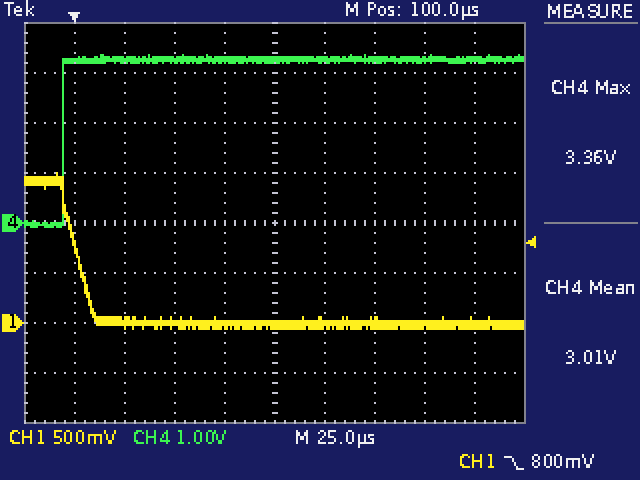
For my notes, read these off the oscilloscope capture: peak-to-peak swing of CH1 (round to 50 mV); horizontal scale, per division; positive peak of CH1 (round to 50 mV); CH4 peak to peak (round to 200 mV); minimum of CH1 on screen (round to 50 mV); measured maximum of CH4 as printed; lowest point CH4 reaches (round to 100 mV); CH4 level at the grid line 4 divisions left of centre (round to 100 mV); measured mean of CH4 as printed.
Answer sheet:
1.55 V
25 µs
1.50 V
3.4 V
-50 mV
3.36 V
-100 mV
3.2 V
3.01 V
